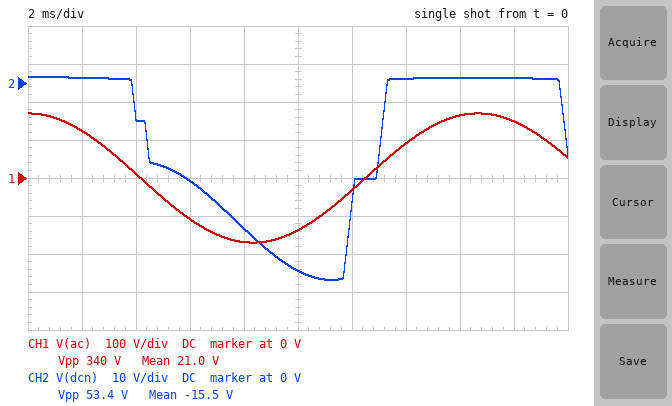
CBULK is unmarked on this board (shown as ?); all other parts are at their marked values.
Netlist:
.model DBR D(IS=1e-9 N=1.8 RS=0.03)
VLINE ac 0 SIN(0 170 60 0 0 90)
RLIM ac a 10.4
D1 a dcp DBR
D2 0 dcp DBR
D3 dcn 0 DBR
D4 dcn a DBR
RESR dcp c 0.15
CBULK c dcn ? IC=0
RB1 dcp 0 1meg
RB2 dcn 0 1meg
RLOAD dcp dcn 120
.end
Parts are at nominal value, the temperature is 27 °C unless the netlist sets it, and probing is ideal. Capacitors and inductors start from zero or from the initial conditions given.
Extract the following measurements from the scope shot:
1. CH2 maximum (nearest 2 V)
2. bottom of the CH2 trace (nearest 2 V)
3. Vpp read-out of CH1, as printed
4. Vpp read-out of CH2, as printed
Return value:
2 V
-52 V
340 V
53.4 V
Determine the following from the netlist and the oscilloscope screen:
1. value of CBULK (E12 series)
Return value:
1.8 mF
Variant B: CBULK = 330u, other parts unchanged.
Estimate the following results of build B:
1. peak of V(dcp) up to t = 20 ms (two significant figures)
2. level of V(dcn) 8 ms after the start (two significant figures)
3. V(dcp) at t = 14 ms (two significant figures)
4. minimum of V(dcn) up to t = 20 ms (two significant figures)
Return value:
130 V
-100 V
91 V
-120 V
